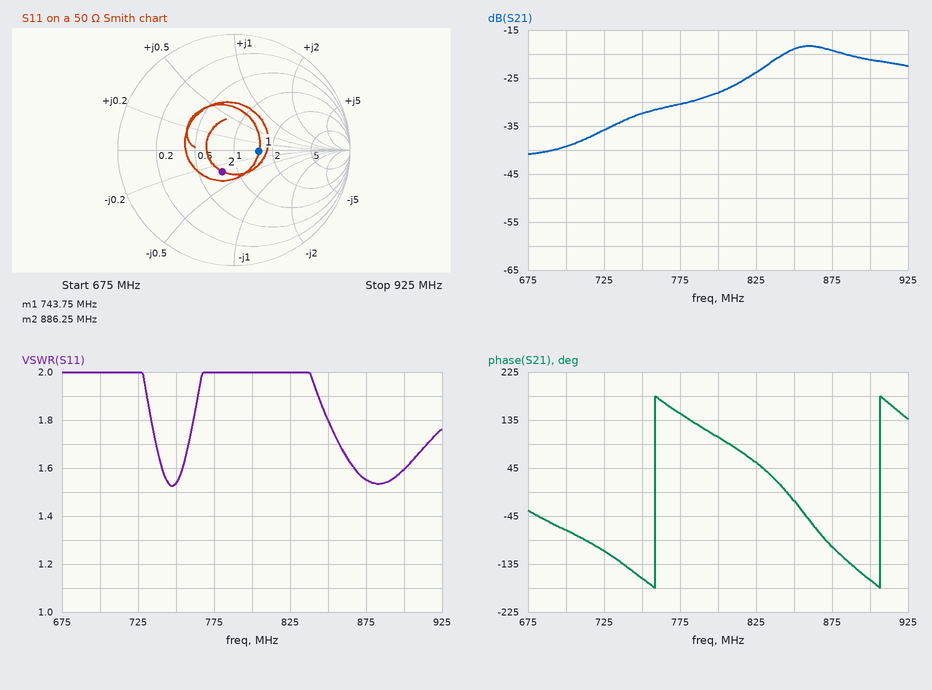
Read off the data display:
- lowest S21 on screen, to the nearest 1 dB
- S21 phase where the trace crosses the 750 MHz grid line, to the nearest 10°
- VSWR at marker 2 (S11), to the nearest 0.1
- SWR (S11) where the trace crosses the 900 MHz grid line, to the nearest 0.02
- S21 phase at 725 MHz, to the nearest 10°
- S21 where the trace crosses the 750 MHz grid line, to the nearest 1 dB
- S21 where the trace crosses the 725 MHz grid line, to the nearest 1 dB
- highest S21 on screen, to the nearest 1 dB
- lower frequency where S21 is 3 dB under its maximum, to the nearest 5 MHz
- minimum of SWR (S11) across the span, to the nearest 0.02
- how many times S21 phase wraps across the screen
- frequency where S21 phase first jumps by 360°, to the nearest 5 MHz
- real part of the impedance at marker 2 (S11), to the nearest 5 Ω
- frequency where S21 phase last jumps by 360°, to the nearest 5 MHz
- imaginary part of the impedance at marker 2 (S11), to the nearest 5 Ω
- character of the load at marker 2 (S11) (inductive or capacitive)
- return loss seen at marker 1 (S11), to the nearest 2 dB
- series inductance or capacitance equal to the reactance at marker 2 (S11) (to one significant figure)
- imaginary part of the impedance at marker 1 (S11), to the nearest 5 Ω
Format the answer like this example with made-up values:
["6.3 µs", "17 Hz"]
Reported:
["-41 dB", "-160°", "1.5", "1.60", "-110°", "-32 dB", "-36 dB", "-18 dB", "835 MHz", "1.52", "2", "760 MHz", "40 Ω", "905 MHz", "-15 Ω", "capacitive", "14 dB", "10 pF", "0 Ω"]
